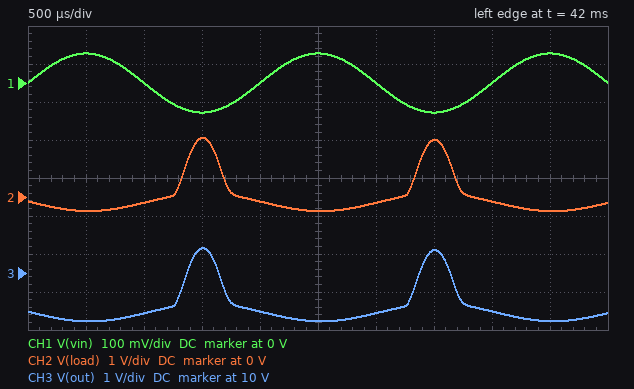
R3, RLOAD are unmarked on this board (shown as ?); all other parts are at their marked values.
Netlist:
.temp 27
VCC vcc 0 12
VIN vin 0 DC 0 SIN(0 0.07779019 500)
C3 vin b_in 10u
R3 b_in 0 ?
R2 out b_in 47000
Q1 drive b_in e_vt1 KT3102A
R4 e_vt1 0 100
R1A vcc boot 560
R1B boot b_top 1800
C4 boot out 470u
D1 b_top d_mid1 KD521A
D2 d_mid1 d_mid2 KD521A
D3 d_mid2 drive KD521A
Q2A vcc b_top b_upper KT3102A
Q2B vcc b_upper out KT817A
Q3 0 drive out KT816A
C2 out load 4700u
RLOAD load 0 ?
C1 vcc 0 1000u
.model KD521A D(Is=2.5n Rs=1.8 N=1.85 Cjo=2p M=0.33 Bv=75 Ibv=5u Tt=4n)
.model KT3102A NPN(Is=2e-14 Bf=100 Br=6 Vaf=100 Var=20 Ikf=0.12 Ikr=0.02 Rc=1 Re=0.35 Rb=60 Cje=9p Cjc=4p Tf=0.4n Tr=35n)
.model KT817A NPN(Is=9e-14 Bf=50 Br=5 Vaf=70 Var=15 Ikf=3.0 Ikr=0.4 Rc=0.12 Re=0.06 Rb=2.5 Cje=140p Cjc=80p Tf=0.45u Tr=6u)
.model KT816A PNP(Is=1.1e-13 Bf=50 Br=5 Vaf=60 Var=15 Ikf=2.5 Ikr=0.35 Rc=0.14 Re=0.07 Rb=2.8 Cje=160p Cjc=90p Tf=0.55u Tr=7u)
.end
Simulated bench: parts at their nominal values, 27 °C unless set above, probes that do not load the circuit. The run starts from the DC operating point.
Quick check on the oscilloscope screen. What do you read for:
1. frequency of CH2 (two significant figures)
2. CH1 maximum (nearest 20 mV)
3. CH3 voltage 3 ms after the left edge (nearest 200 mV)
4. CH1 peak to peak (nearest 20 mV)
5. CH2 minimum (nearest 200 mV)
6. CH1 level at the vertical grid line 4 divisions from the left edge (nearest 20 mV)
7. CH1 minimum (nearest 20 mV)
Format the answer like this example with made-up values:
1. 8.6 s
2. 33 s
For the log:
1. 500 Hz
2. 80 mV
3. 9.0 V
4. 160 mV
5. -400 mV
6. 0 V
7. -80 mV
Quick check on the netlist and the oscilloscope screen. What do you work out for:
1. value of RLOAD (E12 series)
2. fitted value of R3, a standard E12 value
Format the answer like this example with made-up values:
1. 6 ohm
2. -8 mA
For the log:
1. 6.8 Ω
2. 4.7 kΩ
